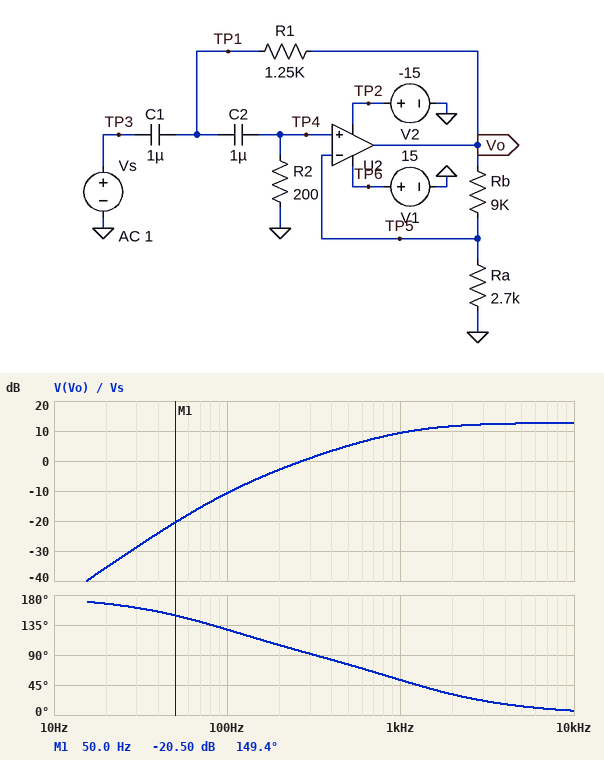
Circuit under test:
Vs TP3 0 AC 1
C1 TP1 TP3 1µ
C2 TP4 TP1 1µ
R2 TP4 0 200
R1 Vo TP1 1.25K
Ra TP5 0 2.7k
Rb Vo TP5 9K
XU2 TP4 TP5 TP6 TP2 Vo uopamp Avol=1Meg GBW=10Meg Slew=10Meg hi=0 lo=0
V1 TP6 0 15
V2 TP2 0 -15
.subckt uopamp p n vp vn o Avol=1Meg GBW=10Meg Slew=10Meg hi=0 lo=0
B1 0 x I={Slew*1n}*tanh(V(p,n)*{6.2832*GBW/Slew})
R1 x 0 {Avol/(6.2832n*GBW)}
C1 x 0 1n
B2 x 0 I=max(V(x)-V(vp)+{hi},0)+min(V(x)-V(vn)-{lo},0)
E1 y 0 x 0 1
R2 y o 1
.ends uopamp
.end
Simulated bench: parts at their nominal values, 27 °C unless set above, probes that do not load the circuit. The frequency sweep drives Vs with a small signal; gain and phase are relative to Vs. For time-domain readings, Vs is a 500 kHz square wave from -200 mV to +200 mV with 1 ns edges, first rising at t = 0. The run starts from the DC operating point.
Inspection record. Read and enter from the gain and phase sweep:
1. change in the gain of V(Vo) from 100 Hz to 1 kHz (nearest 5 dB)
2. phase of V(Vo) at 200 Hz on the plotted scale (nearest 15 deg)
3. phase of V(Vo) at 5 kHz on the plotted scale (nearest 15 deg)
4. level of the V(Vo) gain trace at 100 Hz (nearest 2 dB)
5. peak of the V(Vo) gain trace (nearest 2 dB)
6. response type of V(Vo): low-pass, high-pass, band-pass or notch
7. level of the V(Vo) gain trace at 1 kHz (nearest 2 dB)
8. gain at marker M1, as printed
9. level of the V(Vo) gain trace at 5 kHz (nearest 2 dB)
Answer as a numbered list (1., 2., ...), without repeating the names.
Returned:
1. 20 dB
2. 105 deg
3. 15 deg
4. -10 dB
5. 12 dB
6. high-pass
7. 10 dB
8. -20.50 dB
9. 12 dB
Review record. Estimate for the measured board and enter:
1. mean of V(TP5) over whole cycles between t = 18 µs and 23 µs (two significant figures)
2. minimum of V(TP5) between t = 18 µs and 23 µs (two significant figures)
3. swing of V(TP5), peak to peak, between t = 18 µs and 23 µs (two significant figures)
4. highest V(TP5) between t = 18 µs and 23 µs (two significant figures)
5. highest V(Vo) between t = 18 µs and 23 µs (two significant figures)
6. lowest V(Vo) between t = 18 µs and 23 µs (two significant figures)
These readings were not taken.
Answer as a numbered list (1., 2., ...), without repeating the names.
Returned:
1. 170 mV
2. -30 mV
3. 400 mV
4. 370 mV
5. 1.6 V
6. -130 mV
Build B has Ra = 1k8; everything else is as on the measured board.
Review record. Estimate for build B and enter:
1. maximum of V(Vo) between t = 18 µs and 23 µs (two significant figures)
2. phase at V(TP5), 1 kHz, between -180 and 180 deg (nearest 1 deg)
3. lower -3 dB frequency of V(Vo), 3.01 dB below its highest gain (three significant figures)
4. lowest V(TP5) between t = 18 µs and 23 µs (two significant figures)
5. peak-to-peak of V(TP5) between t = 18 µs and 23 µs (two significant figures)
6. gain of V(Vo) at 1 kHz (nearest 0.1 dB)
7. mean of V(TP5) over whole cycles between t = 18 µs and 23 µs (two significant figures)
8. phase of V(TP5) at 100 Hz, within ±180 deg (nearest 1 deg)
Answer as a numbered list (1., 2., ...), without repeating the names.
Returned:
1. 2.3 V
2. 47 deg
3. 849 Hz
4. -25 mV
5. 400 mV
6. 13.2 dB
7. 180 mV
8. 134 deg
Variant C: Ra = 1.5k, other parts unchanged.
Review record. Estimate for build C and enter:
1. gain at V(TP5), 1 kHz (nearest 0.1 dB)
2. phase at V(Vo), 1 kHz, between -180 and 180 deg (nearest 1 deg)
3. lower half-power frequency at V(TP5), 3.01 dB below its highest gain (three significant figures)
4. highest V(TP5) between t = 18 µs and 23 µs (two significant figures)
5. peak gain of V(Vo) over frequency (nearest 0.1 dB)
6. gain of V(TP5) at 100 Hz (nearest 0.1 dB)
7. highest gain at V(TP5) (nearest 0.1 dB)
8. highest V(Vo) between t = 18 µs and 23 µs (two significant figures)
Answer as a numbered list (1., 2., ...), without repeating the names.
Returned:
1. -1.7 dB
2. 43 deg
3. 708 Hz
4. 380 mV
5. 16.9 dB
6. -21.8 dB
7. 0 dB
8. 2.7 V
